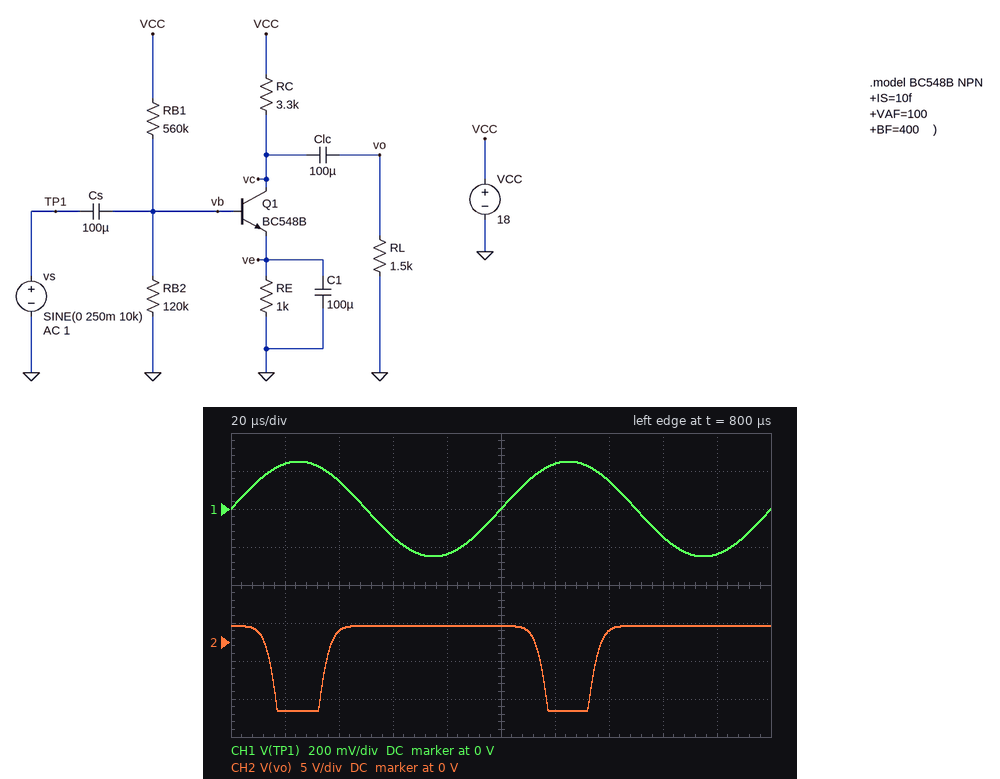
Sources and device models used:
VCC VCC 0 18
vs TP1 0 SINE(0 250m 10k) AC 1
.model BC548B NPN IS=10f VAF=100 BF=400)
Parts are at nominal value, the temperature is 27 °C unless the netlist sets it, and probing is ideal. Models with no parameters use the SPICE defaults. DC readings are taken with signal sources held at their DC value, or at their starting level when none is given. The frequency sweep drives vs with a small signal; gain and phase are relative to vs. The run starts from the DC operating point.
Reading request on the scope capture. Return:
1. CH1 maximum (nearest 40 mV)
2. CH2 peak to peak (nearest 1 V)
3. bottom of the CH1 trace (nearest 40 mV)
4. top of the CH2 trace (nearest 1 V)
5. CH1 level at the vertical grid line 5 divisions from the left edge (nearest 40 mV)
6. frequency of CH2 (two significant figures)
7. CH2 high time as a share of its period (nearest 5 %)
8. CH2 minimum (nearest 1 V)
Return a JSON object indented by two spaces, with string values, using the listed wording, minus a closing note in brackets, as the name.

{
  "CH1 maximum": "240 mV",
  "CH2 peak to peak": "11 V",
  "bottom of the CH1 trace": "-240 mV",
  "top of the CH2 trace": "2 V",
  "CH1 level at the vertical grid line 5 divisions from the left edge": "0 V",
  "frequency of CH2": "10 kHz",
  "CH2 high time as a share of its period": "80 %",
  "CH2 minimum": "-9 V"
}
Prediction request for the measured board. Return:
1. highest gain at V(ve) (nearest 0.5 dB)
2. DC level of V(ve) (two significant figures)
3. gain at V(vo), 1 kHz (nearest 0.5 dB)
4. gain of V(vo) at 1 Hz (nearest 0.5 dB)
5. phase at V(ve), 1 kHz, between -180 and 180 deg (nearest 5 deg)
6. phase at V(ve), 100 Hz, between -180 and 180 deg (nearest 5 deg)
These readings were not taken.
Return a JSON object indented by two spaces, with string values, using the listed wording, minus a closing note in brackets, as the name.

{
  "highest gain at V(ve)": "0 dB",
  "DC level of V(ve)": "2.0 V",
  "gain at V(vo), 1 kHz": "38.0 dB",
  "gain of V(vo) at 1 Hz": "1.0 dB",
  "phase at V(ve), 1 kHz, between -180 and 180 deg": "-85 deg",
  "phase at V(ve), 100 Hz, between -180 and 180 deg": "-40 deg"
}
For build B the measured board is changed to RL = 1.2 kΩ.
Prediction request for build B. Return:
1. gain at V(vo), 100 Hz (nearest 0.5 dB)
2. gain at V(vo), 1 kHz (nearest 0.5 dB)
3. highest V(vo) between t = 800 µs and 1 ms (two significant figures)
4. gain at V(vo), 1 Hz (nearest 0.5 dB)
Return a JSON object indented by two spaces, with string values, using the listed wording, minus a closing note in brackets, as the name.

{
  "gain at V(vo), 100 Hz": "32.5 dB",
  "gain at V(vo), 1 kHz": "36.5 dB",
  "highest V(vo) between t = 800 µs and 1 ms": "1.8 V",
  "gain at V(vo), 1 Hz": "-0.5 dB"
}
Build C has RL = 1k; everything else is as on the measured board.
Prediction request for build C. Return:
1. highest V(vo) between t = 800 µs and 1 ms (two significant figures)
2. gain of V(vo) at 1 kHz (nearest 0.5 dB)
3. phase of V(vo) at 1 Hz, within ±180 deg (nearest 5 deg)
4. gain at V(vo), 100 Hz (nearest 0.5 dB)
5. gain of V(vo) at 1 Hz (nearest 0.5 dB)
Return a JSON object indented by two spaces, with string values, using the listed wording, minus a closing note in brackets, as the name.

{
  "highest V(vo) between t = 800 µs and 1 ms": "1.6 V",
  "gain of V(vo) at 1 kHz": "35.5 dB",
  "phase of V(vo) at 1 Hz, within ±180 deg": "-125 deg",
  "gain at V(vo), 100 Hz": "31.5 dB",
  "gain of V(vo) at 1 Hz": "-1.5 dB"
}
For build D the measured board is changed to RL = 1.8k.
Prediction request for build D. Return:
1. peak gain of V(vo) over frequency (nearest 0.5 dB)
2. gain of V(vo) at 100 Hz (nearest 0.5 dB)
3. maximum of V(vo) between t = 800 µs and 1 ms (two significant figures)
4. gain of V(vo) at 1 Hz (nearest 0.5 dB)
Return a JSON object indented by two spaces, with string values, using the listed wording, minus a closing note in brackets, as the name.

{
  "peak gain of V(vo) over frequency": "39.0 dB",
  "gain of V(vo) at 100 Hz": "35.0 dB",
  "maximum of V(vo) between t = 800 µs and 1 ms": "2.4 V",
  "gain of V(vo) at 1 Hz": "2.0 dB"
}
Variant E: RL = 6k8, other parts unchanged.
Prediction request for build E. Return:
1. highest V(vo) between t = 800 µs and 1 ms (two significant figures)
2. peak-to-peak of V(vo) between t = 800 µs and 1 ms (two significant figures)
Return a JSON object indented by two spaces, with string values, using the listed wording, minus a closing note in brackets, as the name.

{
  "highest V(vo) between t = 800 µs and 1 ms": "4.5 V",
  "peak-to-peak of V(vo) between t = 800 µs and 1 ms": "14 V"
}
